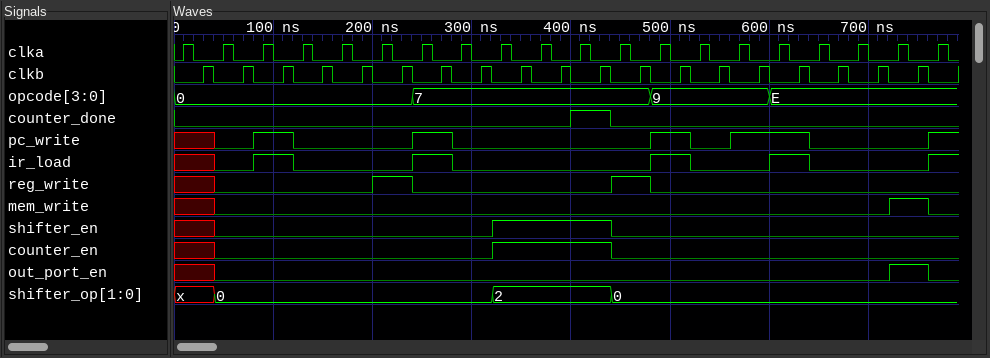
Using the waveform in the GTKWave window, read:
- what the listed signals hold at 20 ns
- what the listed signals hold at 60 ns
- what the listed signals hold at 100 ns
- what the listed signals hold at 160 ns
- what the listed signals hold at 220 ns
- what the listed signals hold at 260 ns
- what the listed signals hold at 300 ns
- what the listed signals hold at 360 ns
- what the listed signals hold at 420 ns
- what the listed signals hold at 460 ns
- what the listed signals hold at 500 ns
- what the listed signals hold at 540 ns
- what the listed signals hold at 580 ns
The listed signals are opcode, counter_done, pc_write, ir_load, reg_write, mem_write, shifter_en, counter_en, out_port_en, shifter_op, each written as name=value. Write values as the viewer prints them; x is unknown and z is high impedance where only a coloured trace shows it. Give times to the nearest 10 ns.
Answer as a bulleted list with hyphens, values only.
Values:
- opcode=0, counter_done=0, pc_write=x, ir_load=x, reg_write=x, mem_write=x, shifter_en=x, counter_en=x, out_port_en=x, shifter_op=x
- opcode=0, counter_done=0, pc_write=0, ir_load=0, reg_write=0, mem_write=0, shifter_en=0, counter_en=0, out_port_en=0, shifter_op=0
- opcode=0, counter_done=0, pc_write=1, ir_load=1, reg_write=0, mem_write=0, shifter_en=0, counter_en=0, out_port_en=0, shifter_op=0
- opcode=0, counter_done=0, pc_write=0, ir_load=0, reg_write=0, mem_write=0, shifter_en=0, counter_en=0, out_port_en=0, shifter_op=0
- opcode=0, counter_done=0, pc_write=0, ir_load=0, reg_write=1, mem_write=0, shifter_en=0, counter_en=0, out_port_en=0, shifter_op=0
- opcode=7, counter_done=0, pc_write=1, ir_load=1, reg_write=0, mem_write=0, shifter_en=0, counter_en=0, out_port_en=0, shifter_op=0
- opcode=7, counter_done=0, pc_write=0, ir_load=0, reg_write=0, mem_write=0, shifter_en=0, counter_en=0, out_port_en=0, shifter_op=0
- opcode=7, counter_done=0, pc_write=0, ir_load=0, reg_write=0, mem_write=0, shifter_en=1, counter_en=1, out_port_en=0, shifter_op=2
- opcode=7, counter_done=1, pc_write=0, ir_load=0, reg_write=0, mem_write=0, shifter_en=1, counter_en=1, out_port_en=0, shifter_op=2
- opcode=7, counter_done=0, pc_write=0, ir_load=0, reg_write=1, mem_write=0, shifter_en=0, counter_en=0, out_port_en=0, shifter_op=0
- opcode=9, counter_done=0, pc_write=1, ir_load=1, reg_write=0, mem_write=0, shifter_en=0, counter_en=0, out_port_en=0, shifter_op=0
- opcode=9, counter_done=0, pc_write=0, ir_load=0, reg_write=0, mem_write=0, shifter_en=0, counter_en=0, out_port_en=0, shifter_op=0
- opcode=9, counter_done=0, pc_write=1, ir_load=0, reg_write=0, mem_write=0, shifter_en=0, counter_en=0, out_port_en=0, shifter_op=0
